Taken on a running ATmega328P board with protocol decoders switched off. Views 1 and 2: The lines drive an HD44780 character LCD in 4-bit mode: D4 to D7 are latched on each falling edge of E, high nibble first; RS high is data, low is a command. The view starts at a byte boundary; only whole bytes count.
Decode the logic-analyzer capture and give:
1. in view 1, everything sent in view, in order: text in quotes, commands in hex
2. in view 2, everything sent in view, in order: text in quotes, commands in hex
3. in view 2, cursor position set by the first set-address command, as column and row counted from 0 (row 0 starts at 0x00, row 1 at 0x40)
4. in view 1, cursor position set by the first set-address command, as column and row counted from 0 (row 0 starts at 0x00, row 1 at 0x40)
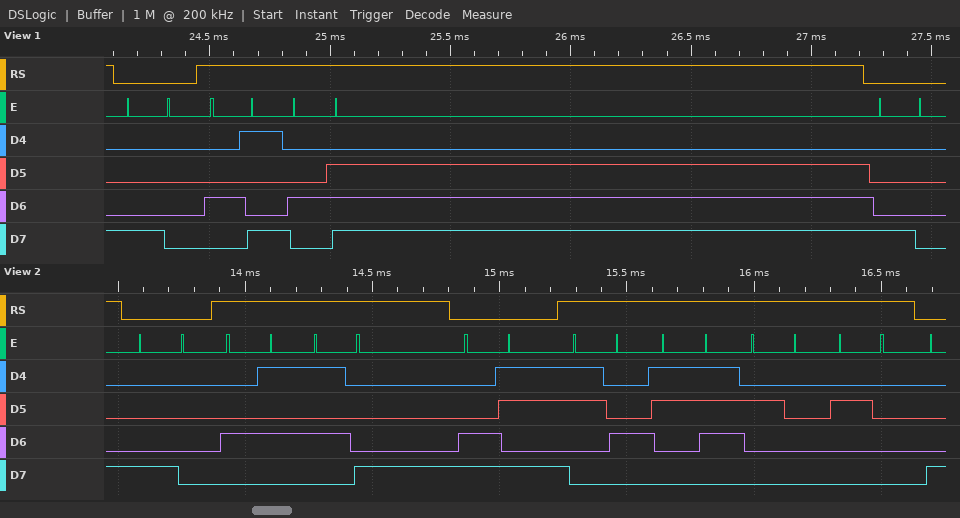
0x80 "IN" 0x80
0x80 "EX" 0xCB "47  "
column 0, row 0
column 0, row 0
